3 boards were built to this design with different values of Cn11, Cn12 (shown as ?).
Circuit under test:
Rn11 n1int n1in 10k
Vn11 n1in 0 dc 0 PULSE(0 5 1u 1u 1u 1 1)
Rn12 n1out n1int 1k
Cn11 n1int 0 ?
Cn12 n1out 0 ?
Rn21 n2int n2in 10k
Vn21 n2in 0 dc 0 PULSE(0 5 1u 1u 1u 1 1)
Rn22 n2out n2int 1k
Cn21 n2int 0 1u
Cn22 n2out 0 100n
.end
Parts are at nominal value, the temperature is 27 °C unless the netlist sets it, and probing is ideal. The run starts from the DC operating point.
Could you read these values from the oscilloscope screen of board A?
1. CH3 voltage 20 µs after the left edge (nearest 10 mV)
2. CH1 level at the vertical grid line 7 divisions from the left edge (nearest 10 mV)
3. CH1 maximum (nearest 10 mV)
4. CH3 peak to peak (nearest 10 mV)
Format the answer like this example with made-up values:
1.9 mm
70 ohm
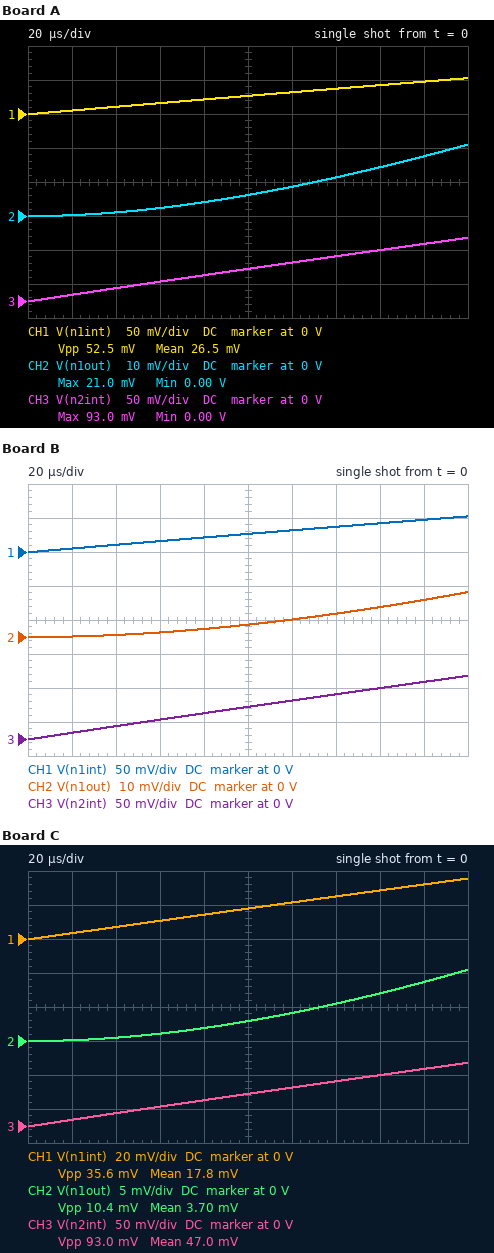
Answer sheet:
10 mV
40 mV
50 mV
90 mV
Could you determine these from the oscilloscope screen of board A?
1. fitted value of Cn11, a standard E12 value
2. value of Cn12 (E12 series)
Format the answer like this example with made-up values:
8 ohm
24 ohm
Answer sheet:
1.8 µF
180 nF
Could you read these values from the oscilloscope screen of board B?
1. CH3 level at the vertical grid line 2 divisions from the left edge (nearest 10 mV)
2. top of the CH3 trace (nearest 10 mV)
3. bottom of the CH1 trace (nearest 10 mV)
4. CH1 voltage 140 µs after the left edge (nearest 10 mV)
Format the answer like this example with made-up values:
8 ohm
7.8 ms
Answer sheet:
20 mV
90 mV
0 V
40 mV
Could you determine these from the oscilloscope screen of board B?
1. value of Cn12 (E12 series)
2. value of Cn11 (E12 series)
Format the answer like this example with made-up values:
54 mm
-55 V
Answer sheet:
330 nF
1.8 µF
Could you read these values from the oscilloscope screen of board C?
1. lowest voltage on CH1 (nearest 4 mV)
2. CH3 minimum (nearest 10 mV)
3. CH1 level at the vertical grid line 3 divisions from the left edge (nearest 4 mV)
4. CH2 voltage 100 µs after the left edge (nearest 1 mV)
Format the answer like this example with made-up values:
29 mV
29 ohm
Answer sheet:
0 V
0 V
12 mV
3 mV
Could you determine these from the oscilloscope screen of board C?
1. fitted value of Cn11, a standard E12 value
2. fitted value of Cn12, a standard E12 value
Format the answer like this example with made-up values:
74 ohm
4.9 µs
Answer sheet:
2.7 µF
270 nF
